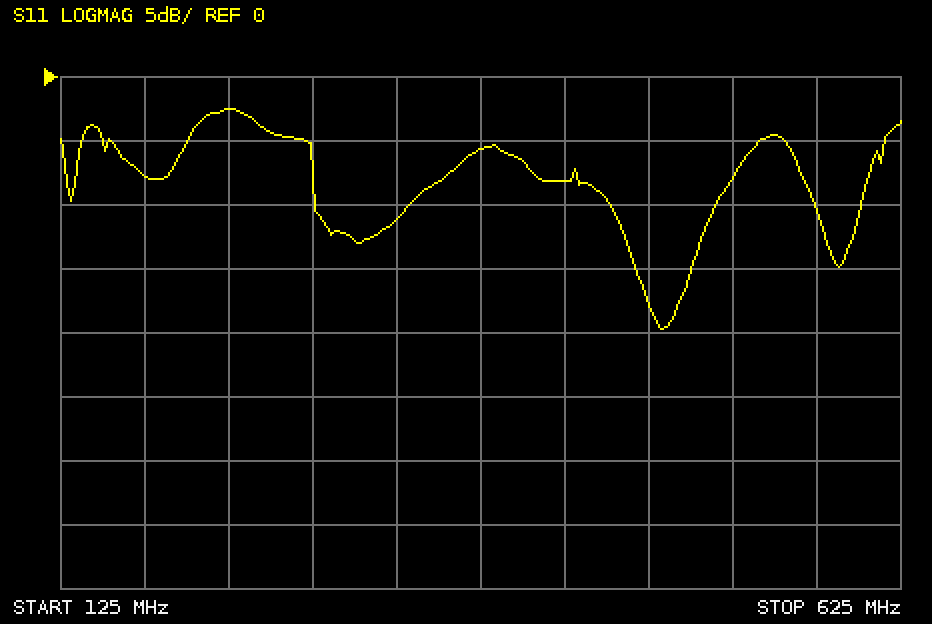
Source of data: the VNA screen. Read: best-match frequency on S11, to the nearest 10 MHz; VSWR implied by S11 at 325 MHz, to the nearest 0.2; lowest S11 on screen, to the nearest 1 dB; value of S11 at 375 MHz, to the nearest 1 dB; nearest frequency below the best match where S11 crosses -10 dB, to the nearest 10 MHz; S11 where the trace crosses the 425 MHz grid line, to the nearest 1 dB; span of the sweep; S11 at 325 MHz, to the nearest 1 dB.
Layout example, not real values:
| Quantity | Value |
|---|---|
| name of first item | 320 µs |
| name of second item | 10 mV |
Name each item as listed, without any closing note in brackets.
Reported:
| Quantity | Value |
|---|---|
| best-match frequency on S11, to the nearest 10 MHz | 480 MHz |
| VSWR implied by S11 at 325 MHz, to the nearest 0.2 | 1.8 |
| lowest S11 on screen, to the nearest 1 dB | -20 dB |
| value of S11 at 375 MHz, to the nearest 1 dB | -6 dB |
| nearest frequency below the best match where S11 crosses -10 dB, to the nearest 10 MHz | 450 MHz |
| S11 where the trace crosses the 425 MHz grid line, to the nearest 1 dB | -8 dB |
| span of the sweep | 500 MHz |
| S11 at 325 MHz, to the nearest 1 dB | -11 dB |
